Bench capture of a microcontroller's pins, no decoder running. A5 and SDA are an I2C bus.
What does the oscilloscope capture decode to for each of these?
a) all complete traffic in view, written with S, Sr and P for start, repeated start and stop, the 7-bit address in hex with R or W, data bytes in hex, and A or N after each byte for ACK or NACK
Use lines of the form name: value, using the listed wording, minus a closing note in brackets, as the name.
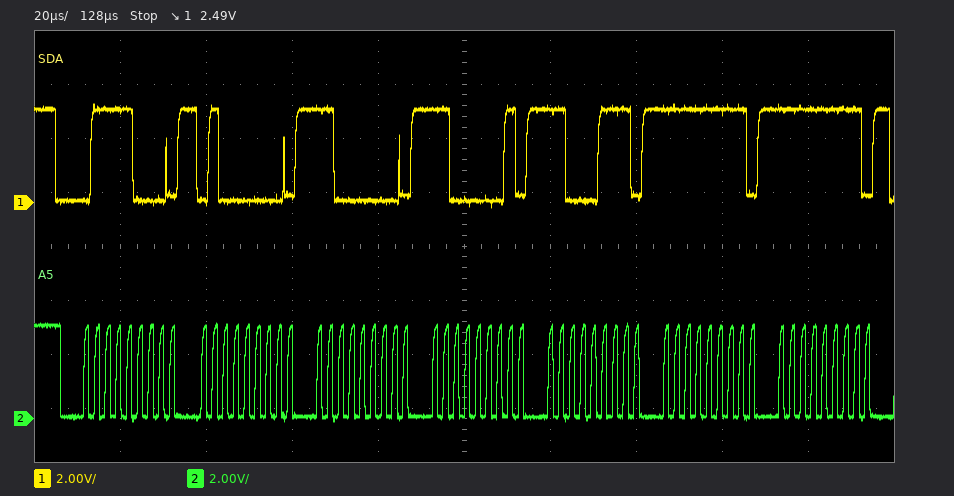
all complete traffic in view, written with S, Sr and P for start, repeated start and stop, the 7-bit address in hex with R or W, data bytes in hex, and A or N after each byte for ACK or NACK: S 3CW A 40 A C0 A C1 A C7 A FF A FF A
